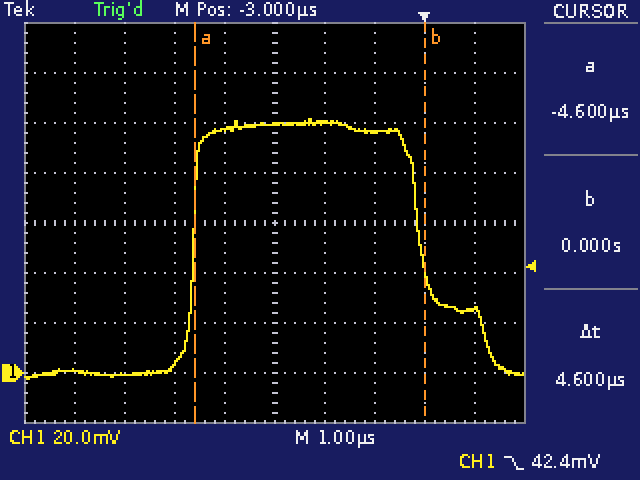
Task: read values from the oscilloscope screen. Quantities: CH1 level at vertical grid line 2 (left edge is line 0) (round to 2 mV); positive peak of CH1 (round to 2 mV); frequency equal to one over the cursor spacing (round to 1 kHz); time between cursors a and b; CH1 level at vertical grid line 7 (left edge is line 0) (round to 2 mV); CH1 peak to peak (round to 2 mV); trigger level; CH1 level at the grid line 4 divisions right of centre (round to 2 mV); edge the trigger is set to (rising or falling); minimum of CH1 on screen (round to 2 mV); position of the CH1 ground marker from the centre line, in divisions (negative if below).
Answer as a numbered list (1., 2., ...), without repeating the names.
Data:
1. 0 mV
2. 102 mV
3. 217 kHz
4. 4.6 µs
5. 96 mV
6. 104 mV
7. 42.4 mV
8. 26 mV
9. falling
10. -2 mV
11. -3.0 div
